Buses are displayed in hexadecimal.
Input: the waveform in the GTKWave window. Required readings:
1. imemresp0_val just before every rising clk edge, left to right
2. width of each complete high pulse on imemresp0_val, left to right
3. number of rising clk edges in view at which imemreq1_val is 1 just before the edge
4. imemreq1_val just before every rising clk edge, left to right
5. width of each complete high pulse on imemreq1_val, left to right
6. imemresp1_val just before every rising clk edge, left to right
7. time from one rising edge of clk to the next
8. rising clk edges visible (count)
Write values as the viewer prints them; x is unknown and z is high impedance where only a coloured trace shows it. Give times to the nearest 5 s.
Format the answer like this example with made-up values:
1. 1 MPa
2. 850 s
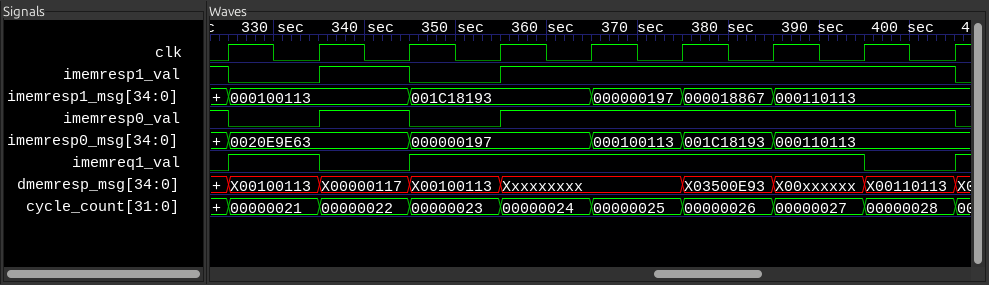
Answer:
1. 1 0 1 0 1 1 1 1 1
2. 10 s, 50 s
3. 6
4. 0 1 0 1 1 1 1 1 0
5. 10 s, 50 s
6. 1 0 1 0 1 1 1 1 1
7. 10 s
8. 9
